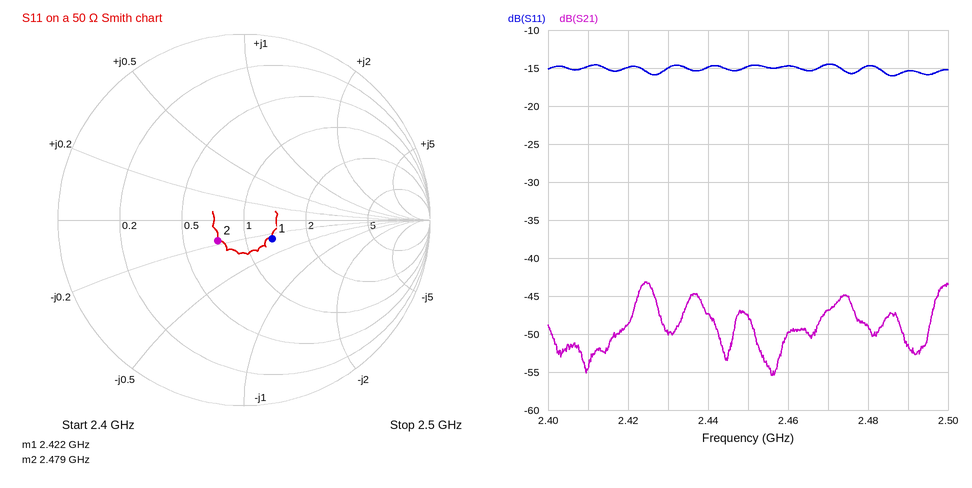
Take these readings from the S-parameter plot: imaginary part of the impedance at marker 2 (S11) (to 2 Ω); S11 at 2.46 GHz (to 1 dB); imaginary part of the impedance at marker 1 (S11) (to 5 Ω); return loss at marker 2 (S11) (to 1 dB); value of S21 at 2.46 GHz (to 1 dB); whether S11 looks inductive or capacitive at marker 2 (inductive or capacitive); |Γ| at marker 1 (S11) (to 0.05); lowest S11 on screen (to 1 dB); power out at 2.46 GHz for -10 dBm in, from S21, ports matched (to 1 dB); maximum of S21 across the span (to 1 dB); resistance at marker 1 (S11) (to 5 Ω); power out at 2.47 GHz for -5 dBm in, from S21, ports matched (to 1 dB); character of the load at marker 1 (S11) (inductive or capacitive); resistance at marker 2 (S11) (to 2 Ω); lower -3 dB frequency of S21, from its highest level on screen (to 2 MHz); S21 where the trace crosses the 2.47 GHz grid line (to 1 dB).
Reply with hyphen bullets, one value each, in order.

- -8 Ω
- -15 dB
- -15 Ω
- 15 dB
- -50 dB
- capacitive
- 0.20
- -16 dB
- -60 dBm
- -43 dB
- 65 Ω
- -52 dBm
- capacitive
- 36 Ω
- 2.422 GHz
- -47 dB
